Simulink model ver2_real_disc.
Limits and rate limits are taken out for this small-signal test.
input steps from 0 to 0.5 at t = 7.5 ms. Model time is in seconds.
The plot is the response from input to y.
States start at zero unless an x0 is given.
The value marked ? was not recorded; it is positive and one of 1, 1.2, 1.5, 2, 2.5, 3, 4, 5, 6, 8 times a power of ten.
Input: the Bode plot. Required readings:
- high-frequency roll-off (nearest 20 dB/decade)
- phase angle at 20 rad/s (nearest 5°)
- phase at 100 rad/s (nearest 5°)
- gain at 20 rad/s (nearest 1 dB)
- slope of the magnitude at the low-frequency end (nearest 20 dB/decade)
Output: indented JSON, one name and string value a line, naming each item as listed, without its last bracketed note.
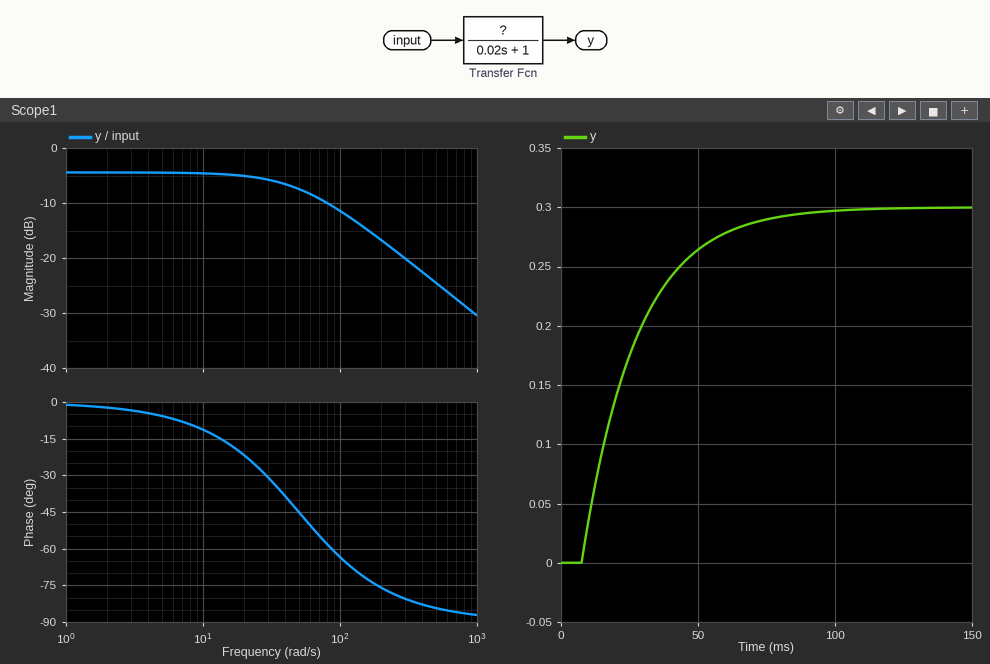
{
  "high-frequency roll-off": "-20 dB/decade",
  "phase angle at 20 rad/s": "-20°",
  "phase at 100 rad/s": "-65°",
  "gain at 20 rad/s": "-5 dB",
  "slope of the magnitude at the low-frequency end": "0 dB/decade"
}
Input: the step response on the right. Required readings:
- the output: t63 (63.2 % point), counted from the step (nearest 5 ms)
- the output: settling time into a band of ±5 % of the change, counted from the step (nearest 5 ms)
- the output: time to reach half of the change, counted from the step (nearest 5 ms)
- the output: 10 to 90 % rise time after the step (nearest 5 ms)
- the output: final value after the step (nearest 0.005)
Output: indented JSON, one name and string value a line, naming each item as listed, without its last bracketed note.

{
  "the output: t63 (63.2 % point), counted from the step": "20 ms",
  "the output: settling time into a band of ±5 % of the change, counted from the step": "60 ms",
  "the output: time to reach half of the change, counted from the step": "15 ms",
  "the output: 10 to 90 % rise time after the step": "45 ms",
  "the output: final value after the step": "0.300"
}
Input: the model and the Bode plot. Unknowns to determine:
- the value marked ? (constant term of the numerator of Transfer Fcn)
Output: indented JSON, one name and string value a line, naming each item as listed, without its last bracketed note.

{
  "the value marked ?": "0.6"
}
